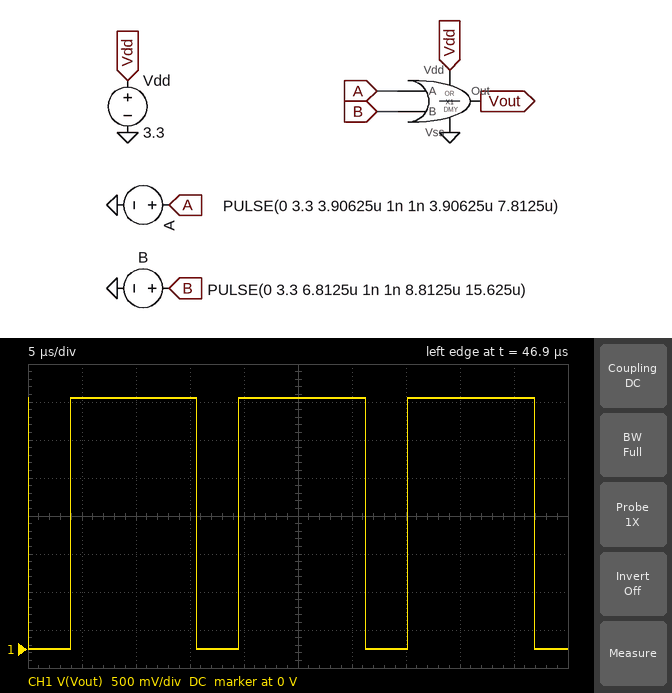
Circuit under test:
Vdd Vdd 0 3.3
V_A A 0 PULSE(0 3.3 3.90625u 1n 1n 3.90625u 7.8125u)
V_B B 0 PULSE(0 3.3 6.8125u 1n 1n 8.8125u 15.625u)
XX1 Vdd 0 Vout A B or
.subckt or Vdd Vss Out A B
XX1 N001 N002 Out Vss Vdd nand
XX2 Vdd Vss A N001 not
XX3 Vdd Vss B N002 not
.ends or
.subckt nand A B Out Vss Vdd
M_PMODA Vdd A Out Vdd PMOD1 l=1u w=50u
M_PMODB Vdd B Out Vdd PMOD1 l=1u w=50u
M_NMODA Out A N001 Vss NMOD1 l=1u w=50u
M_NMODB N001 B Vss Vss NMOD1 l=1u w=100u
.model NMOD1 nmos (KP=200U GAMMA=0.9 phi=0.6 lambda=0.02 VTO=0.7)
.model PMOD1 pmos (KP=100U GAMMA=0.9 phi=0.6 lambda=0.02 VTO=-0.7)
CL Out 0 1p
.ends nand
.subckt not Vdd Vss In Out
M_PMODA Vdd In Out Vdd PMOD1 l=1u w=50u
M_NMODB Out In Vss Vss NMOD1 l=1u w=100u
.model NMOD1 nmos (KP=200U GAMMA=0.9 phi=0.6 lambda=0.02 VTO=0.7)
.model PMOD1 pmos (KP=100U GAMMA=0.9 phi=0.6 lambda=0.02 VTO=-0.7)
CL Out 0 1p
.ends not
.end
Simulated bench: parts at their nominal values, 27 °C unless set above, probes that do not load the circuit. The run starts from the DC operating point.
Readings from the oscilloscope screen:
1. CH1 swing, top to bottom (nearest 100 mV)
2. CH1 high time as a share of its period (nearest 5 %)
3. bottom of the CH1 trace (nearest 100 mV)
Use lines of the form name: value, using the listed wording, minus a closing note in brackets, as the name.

CH1 swing, top to bottom: 3.3 V
CH1 high time as a share of its period: 75 %
bottom of the CH1 trace: 0 V
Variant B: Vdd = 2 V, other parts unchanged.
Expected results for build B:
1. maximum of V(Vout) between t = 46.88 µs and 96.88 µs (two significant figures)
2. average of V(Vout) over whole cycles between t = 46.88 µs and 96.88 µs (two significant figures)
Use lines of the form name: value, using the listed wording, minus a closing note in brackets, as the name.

maximum of V(Vout) between t = 46.88 µs and 96.88 µs: 2.0 V
average of V(Vout) over whole cycles between t = 46.88 µs and 96.88 µs: 1.5 V
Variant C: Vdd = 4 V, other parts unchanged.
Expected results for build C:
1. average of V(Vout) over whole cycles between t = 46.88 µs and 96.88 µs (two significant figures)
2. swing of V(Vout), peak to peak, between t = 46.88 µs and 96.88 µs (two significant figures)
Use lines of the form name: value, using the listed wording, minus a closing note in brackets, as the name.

average of V(Vout) over whole cycles between t = 46.88 µs and 96.88 µs: 3.0 V
swing of V(Vout), peak to peak, between t = 46.88 µs and 96.88 µs: 4.0 V
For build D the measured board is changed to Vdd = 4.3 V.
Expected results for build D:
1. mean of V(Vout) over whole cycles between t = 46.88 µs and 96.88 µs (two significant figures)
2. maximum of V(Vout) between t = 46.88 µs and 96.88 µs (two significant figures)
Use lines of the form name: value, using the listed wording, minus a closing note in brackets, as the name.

mean of V(Vout) over whole cycles between t = 46.88 µs and 96.88 µs: 3.2 V
maximum of V(Vout) between t = 46.88 µs and 96.88 µs: 4.3 V
